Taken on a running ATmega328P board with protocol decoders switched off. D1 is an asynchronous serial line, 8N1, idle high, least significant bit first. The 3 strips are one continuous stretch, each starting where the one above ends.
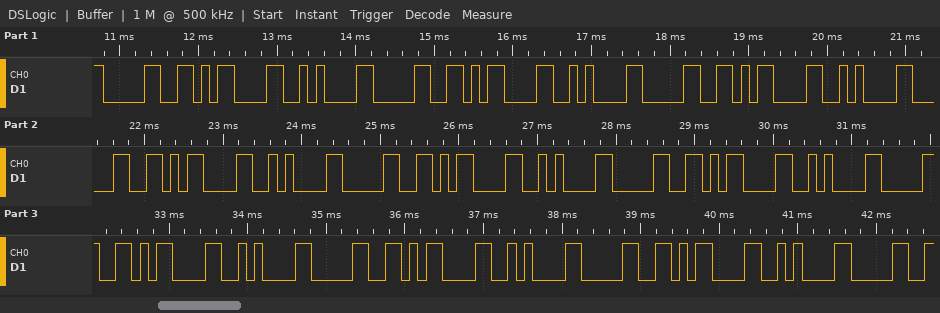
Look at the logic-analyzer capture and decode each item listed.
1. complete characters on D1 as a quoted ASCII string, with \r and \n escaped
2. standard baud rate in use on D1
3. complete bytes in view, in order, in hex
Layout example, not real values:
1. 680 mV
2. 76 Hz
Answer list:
1. "0\r\n0\r\n0\r\n0\r\n0\r\n0\r\n0\r\n0\r\n0\r\n0"
2. 9600 baud
3. 0x30 0x0D 0x0A 0x30 0x0D 0x0A 0x30 0x0D 0x0A 0x30 0x0D 0x0A 0x30 0x0D 0x0A 0x30 0x0D 0x0A 0x30 0x0D 0x0A 0x30 0x0D 0x0A 0x30 0x0D 0x0A 0x30
